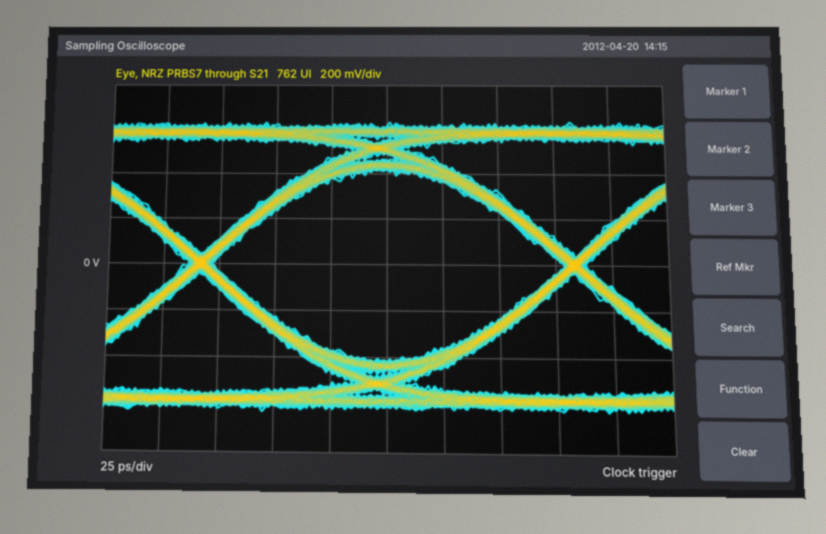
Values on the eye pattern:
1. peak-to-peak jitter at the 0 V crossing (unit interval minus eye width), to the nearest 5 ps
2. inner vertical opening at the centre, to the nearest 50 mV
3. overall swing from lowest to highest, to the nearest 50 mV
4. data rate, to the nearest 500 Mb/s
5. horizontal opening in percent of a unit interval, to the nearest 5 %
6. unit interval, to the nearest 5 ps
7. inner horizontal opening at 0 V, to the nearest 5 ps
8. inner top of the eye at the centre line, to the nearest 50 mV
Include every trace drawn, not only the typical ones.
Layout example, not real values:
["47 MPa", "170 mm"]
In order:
["10 ps", "850 mV", "1.25 V", "6.0 Gb/s", "95 %", "165 ps", "155 ps", "400 mV"]
